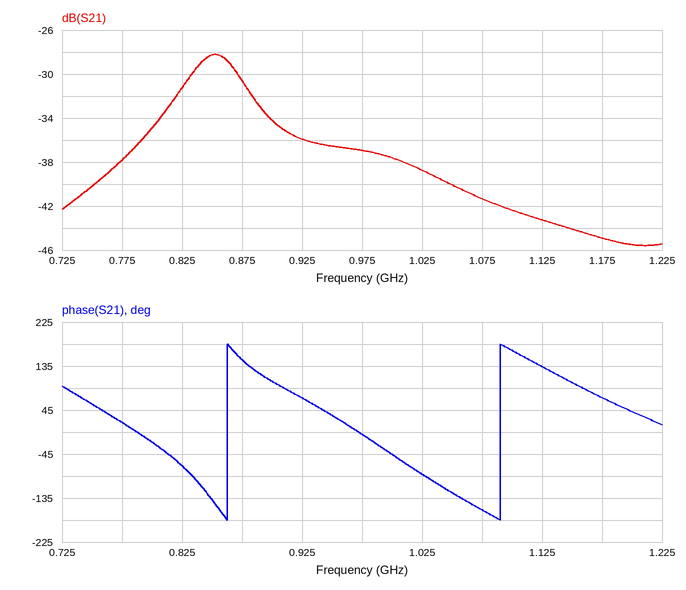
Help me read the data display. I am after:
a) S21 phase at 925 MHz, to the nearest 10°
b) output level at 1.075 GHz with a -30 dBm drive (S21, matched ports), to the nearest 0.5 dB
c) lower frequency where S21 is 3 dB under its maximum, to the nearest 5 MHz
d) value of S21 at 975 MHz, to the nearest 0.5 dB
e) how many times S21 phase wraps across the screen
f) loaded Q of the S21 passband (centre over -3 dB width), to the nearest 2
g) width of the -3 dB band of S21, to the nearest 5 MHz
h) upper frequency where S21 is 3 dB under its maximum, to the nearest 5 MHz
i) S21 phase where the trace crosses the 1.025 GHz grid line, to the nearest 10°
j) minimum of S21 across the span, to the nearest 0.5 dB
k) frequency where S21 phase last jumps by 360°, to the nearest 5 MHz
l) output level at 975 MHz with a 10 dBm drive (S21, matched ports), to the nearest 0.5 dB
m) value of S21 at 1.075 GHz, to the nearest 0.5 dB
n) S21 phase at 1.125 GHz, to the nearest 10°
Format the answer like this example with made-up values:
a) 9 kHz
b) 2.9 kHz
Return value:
a) 70°
b) -71.5 dBm
c) 825 MHz
d) -37.0 dB
e) 2
f) 16
g) 55 MHz
h) 880 MHz
i) -90°
j) -45.5 dB
k) 1.090 GHz
l) -27.0 dBm
m) -41.5 dB
n) 130°
